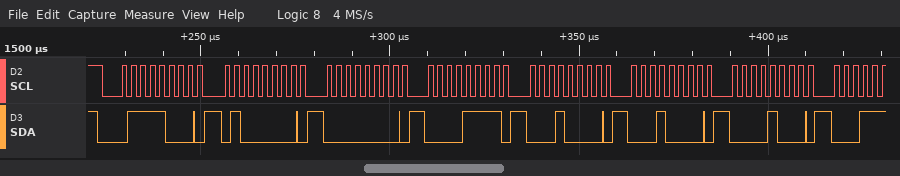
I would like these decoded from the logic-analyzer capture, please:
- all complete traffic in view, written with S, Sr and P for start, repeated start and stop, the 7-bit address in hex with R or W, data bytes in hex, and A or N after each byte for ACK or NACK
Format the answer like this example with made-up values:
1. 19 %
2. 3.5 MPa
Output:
1. S 3CW A 40 A 00 A 0F A 10 A 10 A 08 A
